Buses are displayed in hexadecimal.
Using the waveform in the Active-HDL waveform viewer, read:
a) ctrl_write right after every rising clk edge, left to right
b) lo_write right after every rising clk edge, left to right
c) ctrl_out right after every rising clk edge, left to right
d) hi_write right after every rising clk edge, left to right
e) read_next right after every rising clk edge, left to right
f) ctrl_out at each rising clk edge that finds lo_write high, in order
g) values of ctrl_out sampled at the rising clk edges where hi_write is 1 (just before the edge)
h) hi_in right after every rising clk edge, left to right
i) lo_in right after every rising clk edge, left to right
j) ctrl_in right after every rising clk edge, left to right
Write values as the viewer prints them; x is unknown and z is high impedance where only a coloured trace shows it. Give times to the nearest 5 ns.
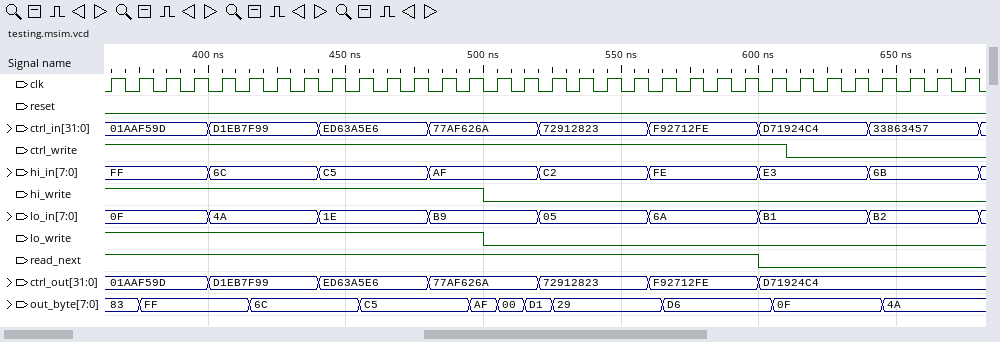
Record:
1 1 1 1 1 1 1 1 1 1 1 1 1 1 1 1 1 1 1 1 1 1 1 1 1 0 0 0 0 0 0 0
1 1 1 1 1 1 1 1 1 1 1 1 1 1 0 0 0 0 0 0 0 0 0 0 0 0 0 0 0 0 0 0
01AAF59D, 01AAF59D, 01AAF59D, 01AAF59D, D1EB7F99, D1EB7F99, D1EB7F99, D1EB7F99, ED63A5E6, ED63A5E6, ED63A5E6, ED63A5E6, 77AF626A, 77AF626A, 77AF626A, 77AF626A, 72912823, 72912823, 72912823, 72912823, F92712FE, F92712FE, F92712FE, F92712FE, D71924C4, D71924C4, D71924C4, D71924C4, D71924C4, D71924C4, D71924C4, D71924C4
1 1 1 1 1 1 1 1 1 1 1 1 1 1 0 0 0 0 0 0 0 0 0 0 0 0 0 0 0 0 0 0
1 1 1 1 1 1 1 1 1 1 1 1 1 1 1 1 1 1 1 1 1 1 1 1 0 0 0 0 0 0 0 0
01AAF59D, 01AAF59D, 01AAF59D, 01AAF59D, D1EB7F99, D1EB7F99, D1EB7F99, D1EB7F99, ED63A5E6, ED63A5E6, ED63A5E6, ED63A5E6, 77AF626A, 77AF626A
01AAF59D, 01AAF59D, 01AAF59D, 01AAF59D, D1EB7F99, D1EB7F99, D1EB7F99, D1EB7F99, ED63A5E6, ED63A5E6, ED63A5E6, ED63A5E6, 77AF626A, 77AF626A
FF, FF, FF, FF, 6C, 6C, 6C, 6C, C5, C5, C5, C5, AF, AF, AF, AF, C2, C2, C2, C2, FE, FE, FE, FE, E3, E3, E3, E3, 6B, 6B, 6B, 6B
0F, 0F, 0F, 0F, 4A, 4A, 4A, 4A, 1E, 1E, 1E, 1E, B9, B9, B9, B9, 05, 05, 05, 05, 6A, 6A, 6A, 6A, B1, B1, B1, B1, B2, B2, B2, B2
01AAF59D, 01AAF59D, 01AAF59D, 01AAF59D, D1EB7F99, D1EB7F99, D1EB7F99, D1EB7F99, ED63A5E6, ED63A5E6, ED63A5E6, ED63A5E6, 77AF626A, 77AF626A, 77AF626A, 77AF626A, 72912823, 72912823, 72912823, 72912823, F92712FE, F92712FE, F92712FE, F92712FE, D71924C4, D71924C4, D71924C4, D71924C4, 33863457, 33863457, 33863457, 33863457
